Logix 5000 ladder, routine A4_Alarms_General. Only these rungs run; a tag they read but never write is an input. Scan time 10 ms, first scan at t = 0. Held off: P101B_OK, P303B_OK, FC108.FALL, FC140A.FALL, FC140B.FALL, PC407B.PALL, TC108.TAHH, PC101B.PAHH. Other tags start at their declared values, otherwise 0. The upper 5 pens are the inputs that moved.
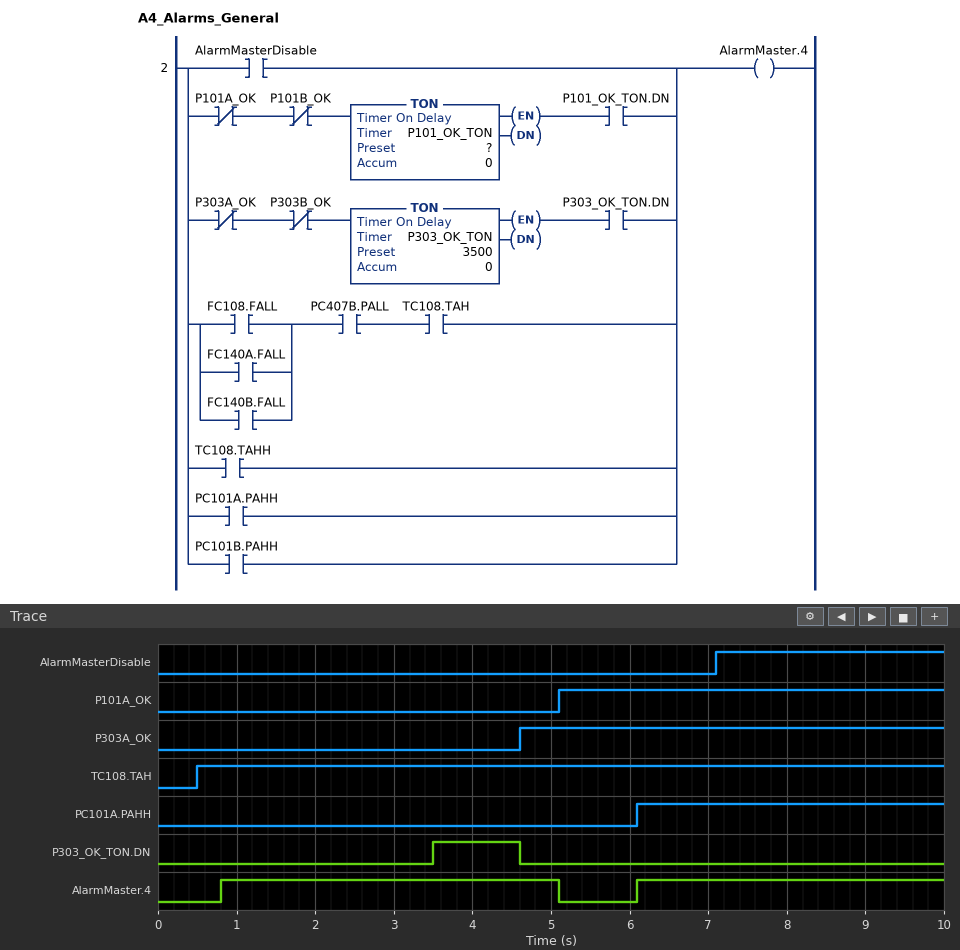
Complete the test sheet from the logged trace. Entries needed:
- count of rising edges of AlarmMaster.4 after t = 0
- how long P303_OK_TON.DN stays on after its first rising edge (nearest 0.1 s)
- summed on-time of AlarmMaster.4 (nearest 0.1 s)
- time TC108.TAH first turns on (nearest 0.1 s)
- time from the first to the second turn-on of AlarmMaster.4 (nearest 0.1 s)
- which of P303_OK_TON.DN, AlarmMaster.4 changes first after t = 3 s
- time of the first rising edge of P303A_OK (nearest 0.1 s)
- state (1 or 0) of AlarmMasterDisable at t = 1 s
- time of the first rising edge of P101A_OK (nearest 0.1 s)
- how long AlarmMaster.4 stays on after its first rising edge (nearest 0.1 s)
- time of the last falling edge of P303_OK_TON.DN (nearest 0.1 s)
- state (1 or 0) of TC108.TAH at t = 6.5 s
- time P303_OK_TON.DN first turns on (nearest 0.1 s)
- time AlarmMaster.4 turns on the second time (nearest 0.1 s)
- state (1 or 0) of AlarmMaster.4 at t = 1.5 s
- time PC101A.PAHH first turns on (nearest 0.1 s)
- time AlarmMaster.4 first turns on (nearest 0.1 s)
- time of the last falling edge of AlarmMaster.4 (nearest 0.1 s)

2
1.1 s
8.2 s
0.5 s
5.3 s
P303_OK_TON.DN
4.6 s
0
5.1 s
4.3 s
4.6 s
1
3.5 s
6.1 s
1
6.1 s
0.8 s
5.1 s
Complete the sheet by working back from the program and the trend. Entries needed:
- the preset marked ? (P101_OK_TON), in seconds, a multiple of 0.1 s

0.8 s
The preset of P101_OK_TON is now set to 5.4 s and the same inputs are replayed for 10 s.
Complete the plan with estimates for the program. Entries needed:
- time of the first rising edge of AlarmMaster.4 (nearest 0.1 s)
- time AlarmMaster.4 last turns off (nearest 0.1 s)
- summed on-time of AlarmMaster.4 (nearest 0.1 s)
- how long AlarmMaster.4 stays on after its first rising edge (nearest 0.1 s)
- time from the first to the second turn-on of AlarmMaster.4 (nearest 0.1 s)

3.5 s
4.6 s
5.0 s
1.1 s
2.6 s
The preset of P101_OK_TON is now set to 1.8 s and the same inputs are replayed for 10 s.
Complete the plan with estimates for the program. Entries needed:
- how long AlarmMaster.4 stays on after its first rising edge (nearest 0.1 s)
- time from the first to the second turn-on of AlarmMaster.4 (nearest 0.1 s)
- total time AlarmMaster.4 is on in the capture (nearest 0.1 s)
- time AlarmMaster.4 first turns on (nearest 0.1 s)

3.3 s
4.3 s
7.2 s
1.8 s
